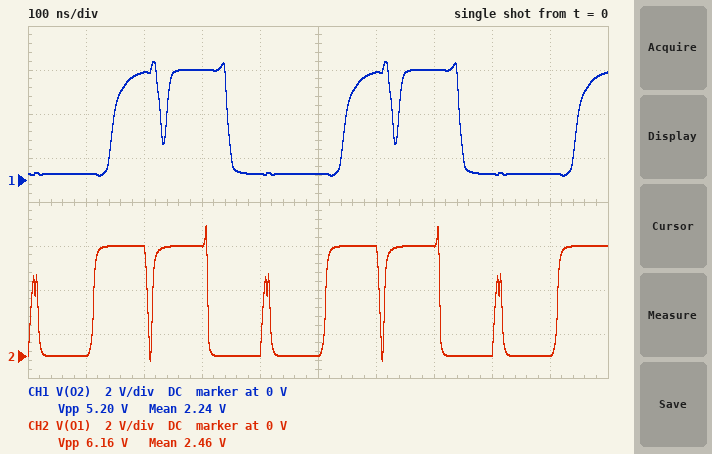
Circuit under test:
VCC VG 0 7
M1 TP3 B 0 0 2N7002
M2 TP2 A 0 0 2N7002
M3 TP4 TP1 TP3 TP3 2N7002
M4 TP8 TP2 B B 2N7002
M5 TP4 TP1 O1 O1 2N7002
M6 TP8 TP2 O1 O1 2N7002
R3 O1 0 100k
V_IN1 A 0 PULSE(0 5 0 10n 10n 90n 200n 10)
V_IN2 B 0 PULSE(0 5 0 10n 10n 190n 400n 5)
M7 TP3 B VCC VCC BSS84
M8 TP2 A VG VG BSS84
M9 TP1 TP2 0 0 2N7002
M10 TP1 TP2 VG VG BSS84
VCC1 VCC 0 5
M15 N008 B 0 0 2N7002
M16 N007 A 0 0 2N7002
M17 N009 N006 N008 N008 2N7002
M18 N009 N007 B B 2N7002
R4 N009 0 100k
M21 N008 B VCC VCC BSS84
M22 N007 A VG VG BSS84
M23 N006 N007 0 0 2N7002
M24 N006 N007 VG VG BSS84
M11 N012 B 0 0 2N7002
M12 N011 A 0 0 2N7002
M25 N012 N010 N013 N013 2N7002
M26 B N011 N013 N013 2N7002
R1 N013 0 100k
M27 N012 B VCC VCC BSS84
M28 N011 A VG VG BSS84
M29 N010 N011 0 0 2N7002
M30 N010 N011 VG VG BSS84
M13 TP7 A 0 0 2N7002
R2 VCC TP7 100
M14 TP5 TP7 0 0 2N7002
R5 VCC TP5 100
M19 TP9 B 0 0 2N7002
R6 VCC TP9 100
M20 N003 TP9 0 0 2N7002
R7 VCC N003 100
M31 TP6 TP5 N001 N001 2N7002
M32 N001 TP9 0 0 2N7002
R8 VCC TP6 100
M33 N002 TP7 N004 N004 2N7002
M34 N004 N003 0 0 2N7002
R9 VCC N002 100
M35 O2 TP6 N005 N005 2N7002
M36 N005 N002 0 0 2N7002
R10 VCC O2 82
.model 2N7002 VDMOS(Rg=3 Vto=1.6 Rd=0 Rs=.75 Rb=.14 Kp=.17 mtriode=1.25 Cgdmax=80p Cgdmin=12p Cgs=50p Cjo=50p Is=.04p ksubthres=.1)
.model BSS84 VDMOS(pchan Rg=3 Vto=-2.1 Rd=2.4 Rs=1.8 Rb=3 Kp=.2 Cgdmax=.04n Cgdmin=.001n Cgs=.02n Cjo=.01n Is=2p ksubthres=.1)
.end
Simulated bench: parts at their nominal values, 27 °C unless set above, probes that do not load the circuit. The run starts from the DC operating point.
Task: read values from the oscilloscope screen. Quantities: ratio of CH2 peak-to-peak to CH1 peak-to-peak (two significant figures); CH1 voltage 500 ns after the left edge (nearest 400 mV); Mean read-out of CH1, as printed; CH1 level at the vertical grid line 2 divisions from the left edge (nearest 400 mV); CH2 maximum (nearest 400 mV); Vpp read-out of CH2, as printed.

1.2
400 mV
2.24 V
4.8 V
6.0 V
6.16 V
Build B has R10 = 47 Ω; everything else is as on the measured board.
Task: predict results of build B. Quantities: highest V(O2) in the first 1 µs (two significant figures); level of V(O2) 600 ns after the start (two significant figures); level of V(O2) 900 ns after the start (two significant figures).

5.3 V
5.0 V
440 mV
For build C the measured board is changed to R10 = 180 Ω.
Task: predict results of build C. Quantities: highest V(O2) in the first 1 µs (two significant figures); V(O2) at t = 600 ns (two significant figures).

5.5 V
4.3 V
